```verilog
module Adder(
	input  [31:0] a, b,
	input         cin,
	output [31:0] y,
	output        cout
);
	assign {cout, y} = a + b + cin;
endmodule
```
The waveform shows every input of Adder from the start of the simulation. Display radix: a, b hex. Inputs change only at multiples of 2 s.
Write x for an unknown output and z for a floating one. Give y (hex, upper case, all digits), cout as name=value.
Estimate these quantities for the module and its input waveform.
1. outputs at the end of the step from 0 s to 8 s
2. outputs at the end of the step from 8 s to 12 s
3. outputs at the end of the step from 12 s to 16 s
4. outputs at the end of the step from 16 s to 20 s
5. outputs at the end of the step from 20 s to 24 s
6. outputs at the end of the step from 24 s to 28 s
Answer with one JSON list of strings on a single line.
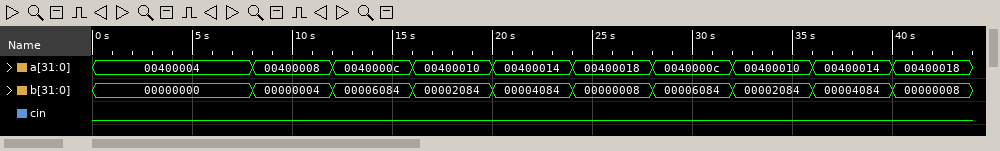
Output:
["y=00400004, cout=0", "y=0040000C, cout=0", "y=00406090, cout=0", "y=00402094, cout=0", "y=00404098, cout=0", "y=00400020, cout=0"]
